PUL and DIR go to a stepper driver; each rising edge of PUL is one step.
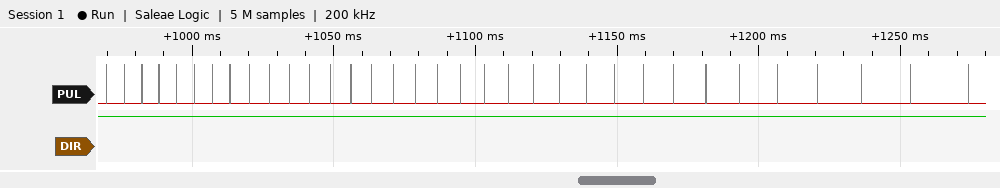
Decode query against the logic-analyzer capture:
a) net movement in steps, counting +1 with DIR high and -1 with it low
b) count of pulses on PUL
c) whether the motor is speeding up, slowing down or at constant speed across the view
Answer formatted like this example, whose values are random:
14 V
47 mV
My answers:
+34
34
slowing down
